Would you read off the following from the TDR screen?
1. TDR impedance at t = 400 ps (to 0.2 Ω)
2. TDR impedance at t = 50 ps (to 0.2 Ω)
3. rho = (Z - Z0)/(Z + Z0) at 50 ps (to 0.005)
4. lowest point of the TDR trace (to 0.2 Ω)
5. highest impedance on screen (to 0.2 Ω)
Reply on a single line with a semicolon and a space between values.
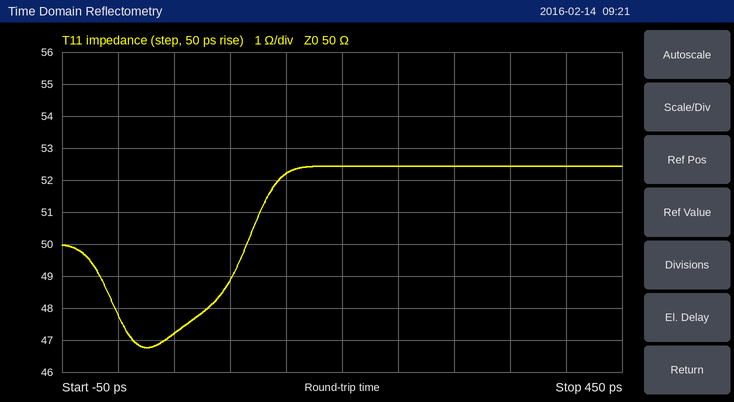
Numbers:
52.4 Ω; 47.2 Ω; -0.030; 46.8 Ω; 52.4 Ω
